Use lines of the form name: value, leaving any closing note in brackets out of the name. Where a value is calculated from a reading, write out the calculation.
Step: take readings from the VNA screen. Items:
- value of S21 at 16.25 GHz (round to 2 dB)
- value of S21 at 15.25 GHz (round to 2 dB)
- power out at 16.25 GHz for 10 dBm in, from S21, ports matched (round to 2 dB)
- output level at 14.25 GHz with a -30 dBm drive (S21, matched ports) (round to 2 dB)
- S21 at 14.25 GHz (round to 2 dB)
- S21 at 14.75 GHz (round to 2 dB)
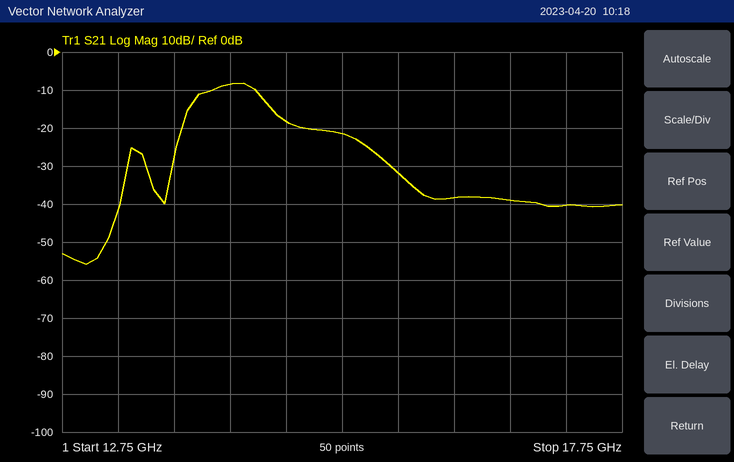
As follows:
value of S21 at 16.25 GHz: -38 dB
value of S21 at 15.25 GHz: -22 dB
power out at 16.25 GHz for 10 dBm in, from S21, ports matched: 10 dBm + (-38 dB) = -28 dBm
output level at 14.25 GHz with a -30 dBm drive (S21, matched ports): -30 dBm + (-8 dB) = -38 dBm
S21 at 14.25 GHz: -8 dB
S21 at 14.75 GHz: -18 dB
